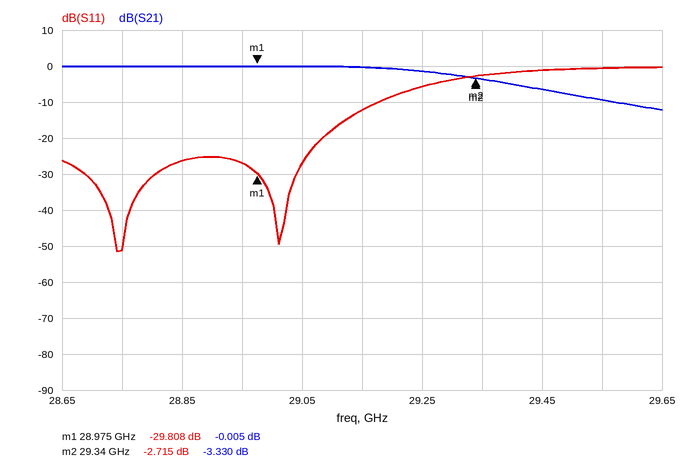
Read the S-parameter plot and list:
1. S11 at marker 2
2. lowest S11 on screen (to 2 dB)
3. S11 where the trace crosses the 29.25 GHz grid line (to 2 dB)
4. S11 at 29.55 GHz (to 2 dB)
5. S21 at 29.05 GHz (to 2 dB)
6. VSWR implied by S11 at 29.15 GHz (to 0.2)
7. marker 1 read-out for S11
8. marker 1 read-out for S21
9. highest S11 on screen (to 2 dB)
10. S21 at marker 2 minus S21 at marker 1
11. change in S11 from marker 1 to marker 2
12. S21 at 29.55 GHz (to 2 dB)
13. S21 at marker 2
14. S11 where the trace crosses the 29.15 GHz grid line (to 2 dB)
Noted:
-2.715 dB
-52 dB
-6 dB
0 dB
0 dB
1.6
-29.808 dB
-0.005 dB
0 dB
-3.325 dB
27.093 dB
-10 dB
-3.330 dB
-12 dB
